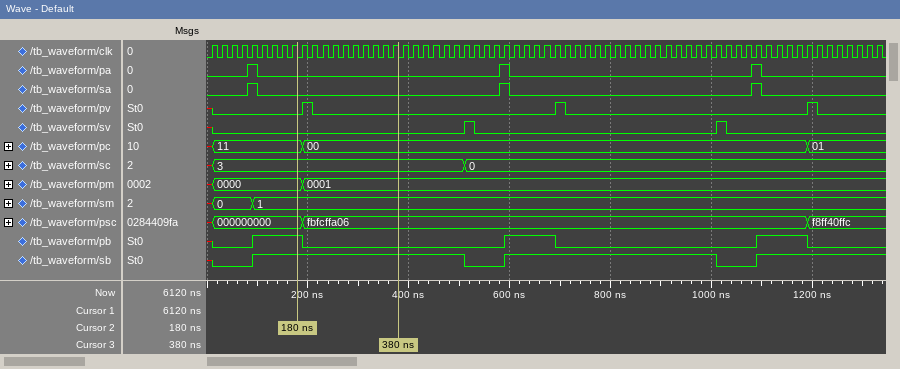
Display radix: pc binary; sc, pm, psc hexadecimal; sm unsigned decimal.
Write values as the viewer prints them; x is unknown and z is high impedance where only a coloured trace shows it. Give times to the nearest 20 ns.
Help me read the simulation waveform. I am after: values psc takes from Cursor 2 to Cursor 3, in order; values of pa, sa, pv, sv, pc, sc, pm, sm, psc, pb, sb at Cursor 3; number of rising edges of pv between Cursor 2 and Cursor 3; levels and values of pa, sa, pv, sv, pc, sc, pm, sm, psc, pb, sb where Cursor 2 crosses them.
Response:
000000000, fbfcffa06
pa=0, sa=0, pv=0, sv=0, pc=00, sc=3, pm=0001, sm=1, psc=fbfcffa06, pb=0, sb=1
1
pa=0, sa=0, pv=0, sv=0, pc=11, sc=3, pm=0000, sm=1, psc=000000000, pb=1, sb=1
